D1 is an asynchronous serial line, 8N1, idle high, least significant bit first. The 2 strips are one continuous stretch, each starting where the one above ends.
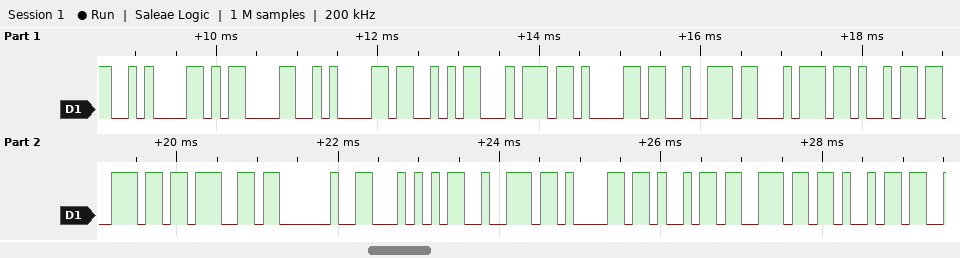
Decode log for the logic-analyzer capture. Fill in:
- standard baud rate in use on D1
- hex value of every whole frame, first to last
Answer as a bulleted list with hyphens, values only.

- 9600 baud
- 0A 0D 0A 53 74 61 72 74 69 6E 67 20 54 72 61 69 6E 69
